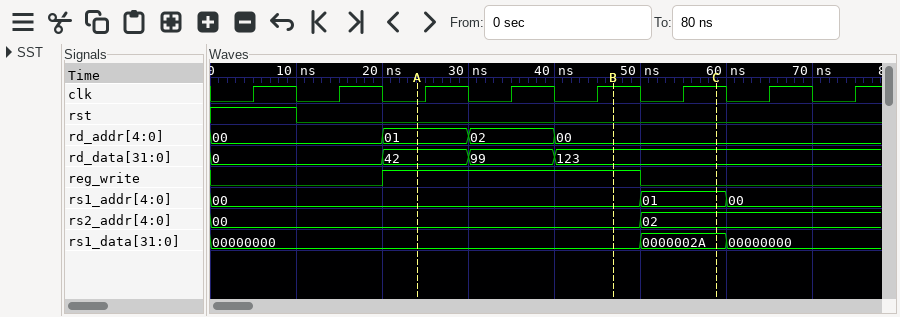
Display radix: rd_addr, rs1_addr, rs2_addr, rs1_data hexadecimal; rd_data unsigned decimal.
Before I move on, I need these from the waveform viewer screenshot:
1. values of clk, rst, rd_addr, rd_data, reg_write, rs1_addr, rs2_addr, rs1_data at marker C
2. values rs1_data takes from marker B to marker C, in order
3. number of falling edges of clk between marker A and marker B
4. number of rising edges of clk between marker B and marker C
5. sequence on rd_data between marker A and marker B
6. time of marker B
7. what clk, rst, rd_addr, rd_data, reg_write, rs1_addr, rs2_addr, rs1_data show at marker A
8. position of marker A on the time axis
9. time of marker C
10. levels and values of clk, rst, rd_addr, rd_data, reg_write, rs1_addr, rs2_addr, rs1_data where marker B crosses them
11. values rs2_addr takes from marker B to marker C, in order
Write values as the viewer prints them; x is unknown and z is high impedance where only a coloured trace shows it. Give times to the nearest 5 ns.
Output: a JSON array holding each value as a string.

["clk=1, rst=0, rd_addr=00, rd_data=123, reg_write=0, rs1_addr=01, rs2_addr=02, rs1_data=0000002A", "00000000, 0000002A", "2", "1", "42, 99, 123", "45 ns", "clk=0, rst=0, rd_addr=01, rd_data=42, reg_write=1, rs1_addr=00, rs2_addr=00, rs1_data=00000000", "25 ns", "60 ns", "clk=1, rst=0, rd_addr=00, rd_data=123, reg_write=1, rs1_addr=00, rs2_addr=00, rs1_data=00000000", "00, 02"]
